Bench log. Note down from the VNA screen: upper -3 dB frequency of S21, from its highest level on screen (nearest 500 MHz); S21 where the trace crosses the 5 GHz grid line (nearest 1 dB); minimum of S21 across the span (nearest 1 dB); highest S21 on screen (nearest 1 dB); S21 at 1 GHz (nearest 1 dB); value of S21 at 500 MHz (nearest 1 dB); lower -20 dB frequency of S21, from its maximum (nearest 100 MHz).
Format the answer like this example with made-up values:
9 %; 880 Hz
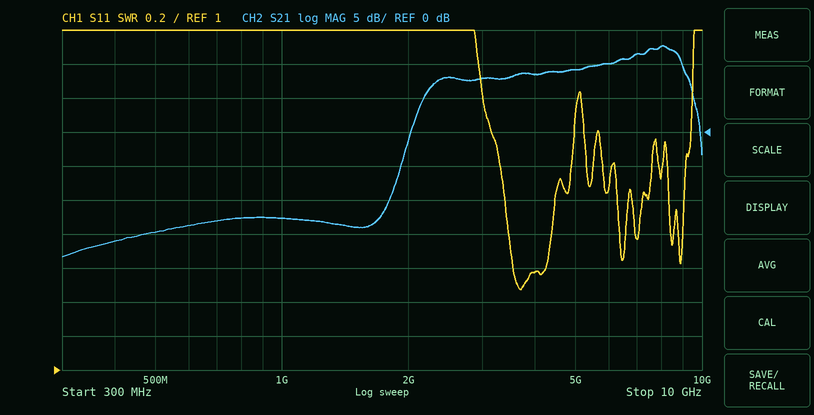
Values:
9.0 GHz; 9 dB; -18 dB; 13 dB; -13 dB; -15 dB; 1.9 GHz
